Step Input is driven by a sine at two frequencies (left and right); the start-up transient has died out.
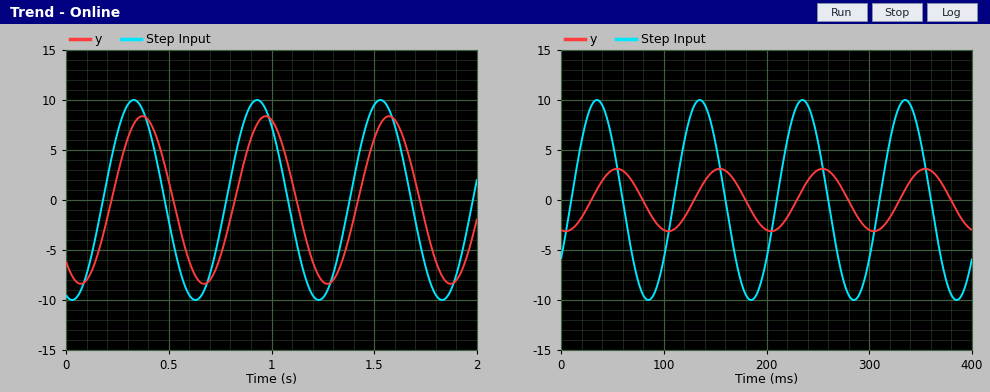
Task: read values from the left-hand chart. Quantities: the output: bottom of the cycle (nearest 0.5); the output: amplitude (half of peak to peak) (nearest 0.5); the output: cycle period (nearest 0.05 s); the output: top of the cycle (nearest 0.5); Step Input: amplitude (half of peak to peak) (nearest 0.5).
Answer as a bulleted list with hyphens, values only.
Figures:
- -8.5
- 8.5
- 0.60 s
- 8.5
- 10.0
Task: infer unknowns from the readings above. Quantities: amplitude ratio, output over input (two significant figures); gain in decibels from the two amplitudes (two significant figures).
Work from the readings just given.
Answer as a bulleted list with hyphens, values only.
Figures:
- 0.85
- -1.4 dB
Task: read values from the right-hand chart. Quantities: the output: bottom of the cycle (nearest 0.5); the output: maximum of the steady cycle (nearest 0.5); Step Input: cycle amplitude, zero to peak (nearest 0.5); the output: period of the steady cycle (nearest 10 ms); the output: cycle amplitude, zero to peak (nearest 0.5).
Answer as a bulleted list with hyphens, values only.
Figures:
- -3.0
- 3.0
- 10.0
- 100 ms
- 3.0
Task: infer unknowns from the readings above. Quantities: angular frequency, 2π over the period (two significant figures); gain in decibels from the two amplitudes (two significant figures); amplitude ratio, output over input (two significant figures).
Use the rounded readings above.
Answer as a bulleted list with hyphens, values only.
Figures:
- 0.063 rad/ms
- -10 dB
- 0.30
